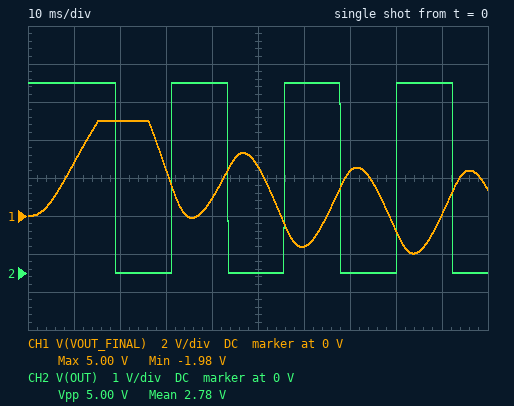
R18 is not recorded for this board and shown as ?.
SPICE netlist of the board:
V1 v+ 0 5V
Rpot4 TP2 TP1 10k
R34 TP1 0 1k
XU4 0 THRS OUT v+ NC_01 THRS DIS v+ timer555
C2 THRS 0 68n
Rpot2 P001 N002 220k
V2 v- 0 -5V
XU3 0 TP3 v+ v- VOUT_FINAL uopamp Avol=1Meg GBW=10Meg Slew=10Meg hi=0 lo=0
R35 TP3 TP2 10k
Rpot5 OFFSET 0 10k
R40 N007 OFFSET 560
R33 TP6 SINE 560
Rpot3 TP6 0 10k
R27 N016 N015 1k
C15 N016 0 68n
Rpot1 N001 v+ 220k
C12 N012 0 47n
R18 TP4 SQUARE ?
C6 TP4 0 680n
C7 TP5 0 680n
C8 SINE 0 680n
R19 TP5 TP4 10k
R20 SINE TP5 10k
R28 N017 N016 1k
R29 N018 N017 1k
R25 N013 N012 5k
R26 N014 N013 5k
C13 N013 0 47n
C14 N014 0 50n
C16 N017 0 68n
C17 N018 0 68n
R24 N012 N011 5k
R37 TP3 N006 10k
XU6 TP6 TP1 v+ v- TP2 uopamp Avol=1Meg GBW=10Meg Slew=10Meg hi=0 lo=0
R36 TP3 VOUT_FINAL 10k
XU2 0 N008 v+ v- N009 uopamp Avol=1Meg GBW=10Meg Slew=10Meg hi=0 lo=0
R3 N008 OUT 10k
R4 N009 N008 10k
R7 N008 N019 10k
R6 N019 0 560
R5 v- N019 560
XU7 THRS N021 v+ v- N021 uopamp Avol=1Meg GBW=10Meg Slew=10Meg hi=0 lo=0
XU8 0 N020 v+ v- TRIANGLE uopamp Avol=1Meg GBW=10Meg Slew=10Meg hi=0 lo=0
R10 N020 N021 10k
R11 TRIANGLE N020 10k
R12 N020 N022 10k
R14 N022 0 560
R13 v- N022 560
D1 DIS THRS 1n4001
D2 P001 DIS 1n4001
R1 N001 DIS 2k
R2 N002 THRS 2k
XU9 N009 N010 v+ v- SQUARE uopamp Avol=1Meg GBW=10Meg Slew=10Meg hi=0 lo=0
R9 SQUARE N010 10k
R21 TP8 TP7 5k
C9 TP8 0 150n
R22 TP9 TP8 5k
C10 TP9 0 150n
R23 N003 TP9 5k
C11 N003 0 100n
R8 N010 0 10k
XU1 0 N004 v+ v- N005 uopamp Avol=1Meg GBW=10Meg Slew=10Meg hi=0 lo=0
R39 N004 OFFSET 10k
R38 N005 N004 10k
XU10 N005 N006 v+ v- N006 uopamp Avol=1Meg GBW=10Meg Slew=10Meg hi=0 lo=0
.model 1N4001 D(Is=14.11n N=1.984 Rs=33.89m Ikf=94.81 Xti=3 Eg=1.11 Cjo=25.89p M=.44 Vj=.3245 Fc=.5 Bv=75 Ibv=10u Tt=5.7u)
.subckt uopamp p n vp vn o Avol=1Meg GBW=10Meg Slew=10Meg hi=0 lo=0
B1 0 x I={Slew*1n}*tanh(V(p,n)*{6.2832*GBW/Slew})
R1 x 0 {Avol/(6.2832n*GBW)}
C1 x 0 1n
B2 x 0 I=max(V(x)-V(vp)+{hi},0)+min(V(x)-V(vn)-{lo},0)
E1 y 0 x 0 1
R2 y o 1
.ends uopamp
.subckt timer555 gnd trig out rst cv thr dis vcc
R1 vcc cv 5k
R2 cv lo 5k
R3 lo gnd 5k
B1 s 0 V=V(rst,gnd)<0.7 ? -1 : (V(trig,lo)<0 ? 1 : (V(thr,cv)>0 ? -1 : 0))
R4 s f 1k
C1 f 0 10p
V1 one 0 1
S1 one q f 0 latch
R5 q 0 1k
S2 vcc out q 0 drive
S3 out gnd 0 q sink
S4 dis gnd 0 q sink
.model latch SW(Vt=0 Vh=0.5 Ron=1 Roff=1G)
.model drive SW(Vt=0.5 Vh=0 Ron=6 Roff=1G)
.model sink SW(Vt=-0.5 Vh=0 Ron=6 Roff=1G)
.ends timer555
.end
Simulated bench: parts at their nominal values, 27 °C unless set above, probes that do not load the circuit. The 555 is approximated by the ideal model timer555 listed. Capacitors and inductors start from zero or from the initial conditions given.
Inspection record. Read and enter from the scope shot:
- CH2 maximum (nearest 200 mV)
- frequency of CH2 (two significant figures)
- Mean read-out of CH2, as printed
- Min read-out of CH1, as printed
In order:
5.0 V
41 Hz
2.78 V
-1.98 V
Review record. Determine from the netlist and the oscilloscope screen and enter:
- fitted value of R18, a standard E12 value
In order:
18 kΩ
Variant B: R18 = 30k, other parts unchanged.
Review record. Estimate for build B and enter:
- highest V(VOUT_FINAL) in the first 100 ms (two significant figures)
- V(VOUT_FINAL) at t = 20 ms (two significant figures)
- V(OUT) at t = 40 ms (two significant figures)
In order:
4.7 V
4.5 V
5.0 V
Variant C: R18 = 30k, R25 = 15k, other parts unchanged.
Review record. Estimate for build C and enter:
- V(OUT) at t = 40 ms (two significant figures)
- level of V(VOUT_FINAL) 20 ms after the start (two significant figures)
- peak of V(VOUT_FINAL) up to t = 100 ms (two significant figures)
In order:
5.0 V
4.5 V
4.7 V
